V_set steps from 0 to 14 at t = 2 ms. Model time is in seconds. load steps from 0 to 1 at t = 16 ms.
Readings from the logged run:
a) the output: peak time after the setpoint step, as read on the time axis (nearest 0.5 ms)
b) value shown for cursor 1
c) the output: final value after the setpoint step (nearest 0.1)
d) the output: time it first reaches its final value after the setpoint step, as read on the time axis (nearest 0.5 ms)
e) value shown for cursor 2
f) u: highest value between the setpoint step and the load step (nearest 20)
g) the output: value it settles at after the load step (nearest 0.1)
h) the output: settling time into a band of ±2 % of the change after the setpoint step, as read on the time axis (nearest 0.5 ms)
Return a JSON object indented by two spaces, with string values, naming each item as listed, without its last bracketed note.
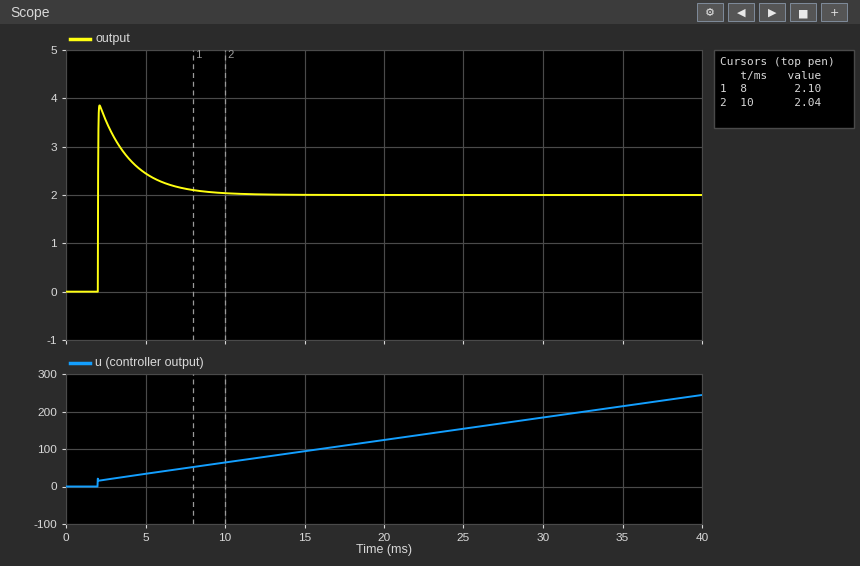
{
  "the output: peak time after the setpoint step, as read on the time axis": "2.0 ms",
  "value shown for cursor 1": "2.10",
  "the output: final value after the setpoint step": "2.0",
  "the output: time it first reaches its final value after the setpoint step, as read on the time axis": "2.0 ms",
  "value shown for cursor 2": "2.04",
  "u: highest value between the setpoint step and the load step": "100",
  "the output: value it settles at after the load step": "2.0",
  "the output: settling time into a band of ±2 % of the change after the setpoint step, as read on the time axis": "10.0 ms"
}
